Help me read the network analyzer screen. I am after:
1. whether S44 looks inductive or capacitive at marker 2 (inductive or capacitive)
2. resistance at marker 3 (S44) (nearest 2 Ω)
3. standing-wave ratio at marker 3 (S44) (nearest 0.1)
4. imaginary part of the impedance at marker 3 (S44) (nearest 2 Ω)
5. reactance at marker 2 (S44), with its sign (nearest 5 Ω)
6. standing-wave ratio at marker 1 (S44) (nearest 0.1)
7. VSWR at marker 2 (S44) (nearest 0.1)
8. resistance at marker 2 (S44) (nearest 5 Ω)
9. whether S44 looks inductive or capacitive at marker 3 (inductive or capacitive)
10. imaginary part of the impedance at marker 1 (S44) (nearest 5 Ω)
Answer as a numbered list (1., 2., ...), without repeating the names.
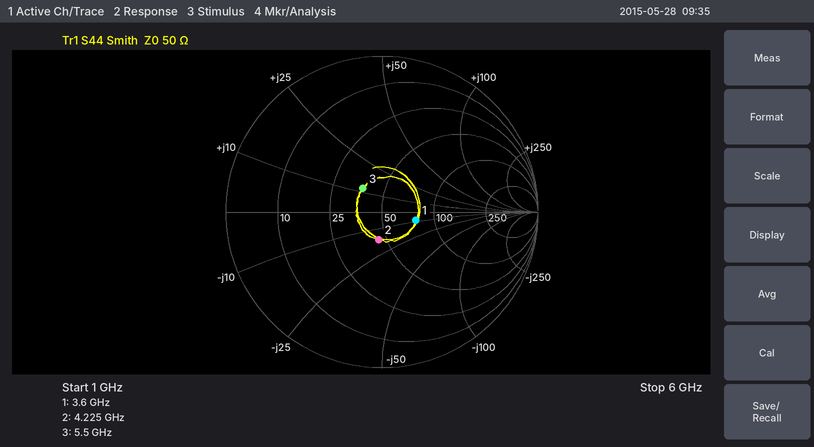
1. capacitive
2. 38 Ω
3. 1.5
4. +12 Ω
5. -15 Ω
6. 1.6
7. 1.4
8. 45 Ω
9. inductive
10. -10 Ω
